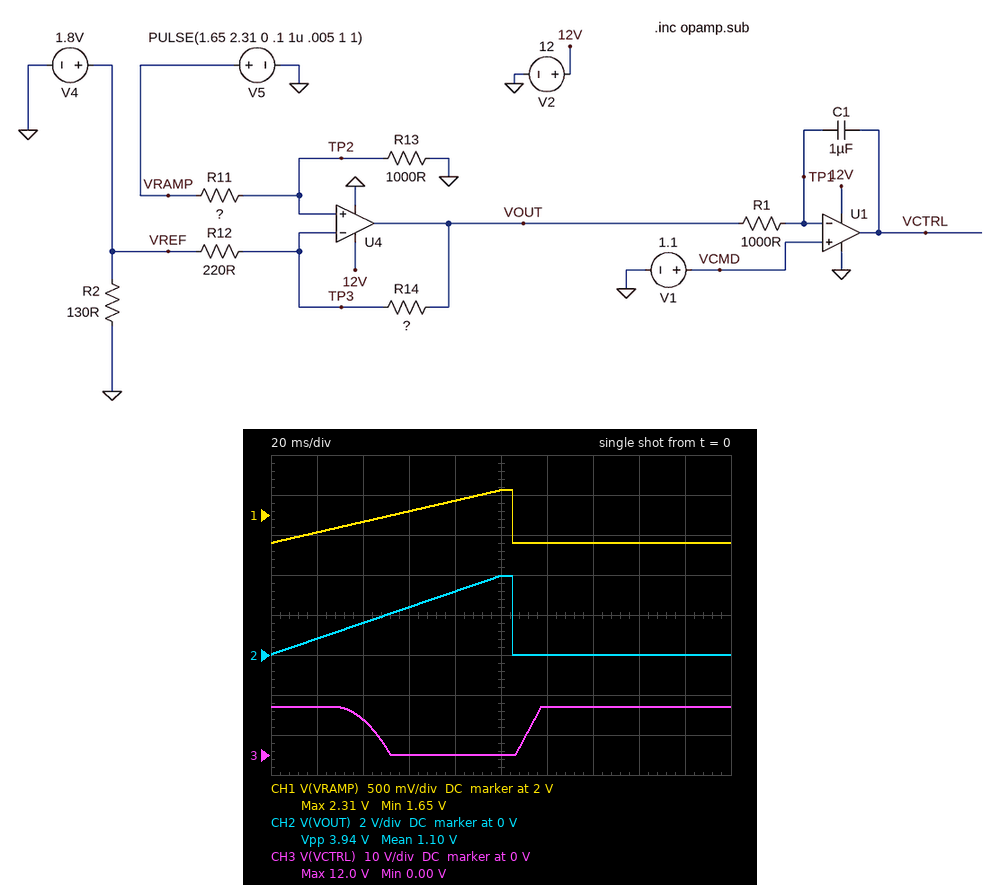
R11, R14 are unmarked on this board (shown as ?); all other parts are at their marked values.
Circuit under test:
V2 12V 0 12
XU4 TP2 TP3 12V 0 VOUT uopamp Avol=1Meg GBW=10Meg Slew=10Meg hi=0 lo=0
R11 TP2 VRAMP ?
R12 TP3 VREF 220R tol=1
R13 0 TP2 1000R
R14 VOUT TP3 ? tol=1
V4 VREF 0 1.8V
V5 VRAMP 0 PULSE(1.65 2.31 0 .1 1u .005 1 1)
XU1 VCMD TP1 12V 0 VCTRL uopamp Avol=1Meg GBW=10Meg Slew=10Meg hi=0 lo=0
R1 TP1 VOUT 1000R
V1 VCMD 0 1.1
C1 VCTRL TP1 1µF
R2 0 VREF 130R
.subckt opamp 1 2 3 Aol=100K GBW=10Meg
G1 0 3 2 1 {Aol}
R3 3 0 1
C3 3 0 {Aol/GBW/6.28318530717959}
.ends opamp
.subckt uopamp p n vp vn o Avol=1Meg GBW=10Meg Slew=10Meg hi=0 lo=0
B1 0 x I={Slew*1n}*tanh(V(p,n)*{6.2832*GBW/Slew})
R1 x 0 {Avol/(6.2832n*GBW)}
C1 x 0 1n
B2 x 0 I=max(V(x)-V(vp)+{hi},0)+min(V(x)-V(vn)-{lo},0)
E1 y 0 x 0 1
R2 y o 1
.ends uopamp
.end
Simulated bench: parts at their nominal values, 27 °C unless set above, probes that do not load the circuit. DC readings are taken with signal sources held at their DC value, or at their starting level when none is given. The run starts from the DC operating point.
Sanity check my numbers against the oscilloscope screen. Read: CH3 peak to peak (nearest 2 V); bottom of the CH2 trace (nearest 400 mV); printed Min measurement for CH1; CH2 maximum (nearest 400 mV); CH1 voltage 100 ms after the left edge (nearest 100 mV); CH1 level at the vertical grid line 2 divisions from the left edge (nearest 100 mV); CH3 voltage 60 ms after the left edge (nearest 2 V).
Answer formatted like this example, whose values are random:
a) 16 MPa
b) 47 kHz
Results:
a) 12 V
b) 0 V
c) 1.65 V
d) 4.0 V
e) 2.3 V
f) 1.9 V
g) 0 V
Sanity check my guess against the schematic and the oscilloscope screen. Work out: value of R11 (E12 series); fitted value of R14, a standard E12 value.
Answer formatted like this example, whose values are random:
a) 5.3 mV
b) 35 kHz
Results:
a) 82 Ω
b) 1.2 kΩ
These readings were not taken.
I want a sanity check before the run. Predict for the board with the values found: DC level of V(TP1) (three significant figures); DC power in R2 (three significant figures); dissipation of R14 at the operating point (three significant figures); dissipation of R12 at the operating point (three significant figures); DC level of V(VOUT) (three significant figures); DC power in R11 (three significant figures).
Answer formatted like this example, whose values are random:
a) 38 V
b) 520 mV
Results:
a) 24.7 mV
b) 24.9 mW
c) 1.88 mW
d) 344 µW
e) 24.7 mV
f) 191 µW
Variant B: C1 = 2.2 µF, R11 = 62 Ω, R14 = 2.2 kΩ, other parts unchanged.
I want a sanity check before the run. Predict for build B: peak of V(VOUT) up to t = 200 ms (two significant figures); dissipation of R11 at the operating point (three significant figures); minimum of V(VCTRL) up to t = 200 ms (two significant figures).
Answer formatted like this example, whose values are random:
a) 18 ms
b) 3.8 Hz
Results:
a) 5.9 V
b) 150 µW
c) -16 mV
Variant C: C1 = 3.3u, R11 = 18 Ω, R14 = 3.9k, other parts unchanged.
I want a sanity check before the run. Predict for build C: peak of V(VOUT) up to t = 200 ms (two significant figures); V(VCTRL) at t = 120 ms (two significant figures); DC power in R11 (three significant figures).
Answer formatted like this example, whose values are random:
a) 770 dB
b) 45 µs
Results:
a) 11 V
b) 2.5 V
c) 47.3 µW
